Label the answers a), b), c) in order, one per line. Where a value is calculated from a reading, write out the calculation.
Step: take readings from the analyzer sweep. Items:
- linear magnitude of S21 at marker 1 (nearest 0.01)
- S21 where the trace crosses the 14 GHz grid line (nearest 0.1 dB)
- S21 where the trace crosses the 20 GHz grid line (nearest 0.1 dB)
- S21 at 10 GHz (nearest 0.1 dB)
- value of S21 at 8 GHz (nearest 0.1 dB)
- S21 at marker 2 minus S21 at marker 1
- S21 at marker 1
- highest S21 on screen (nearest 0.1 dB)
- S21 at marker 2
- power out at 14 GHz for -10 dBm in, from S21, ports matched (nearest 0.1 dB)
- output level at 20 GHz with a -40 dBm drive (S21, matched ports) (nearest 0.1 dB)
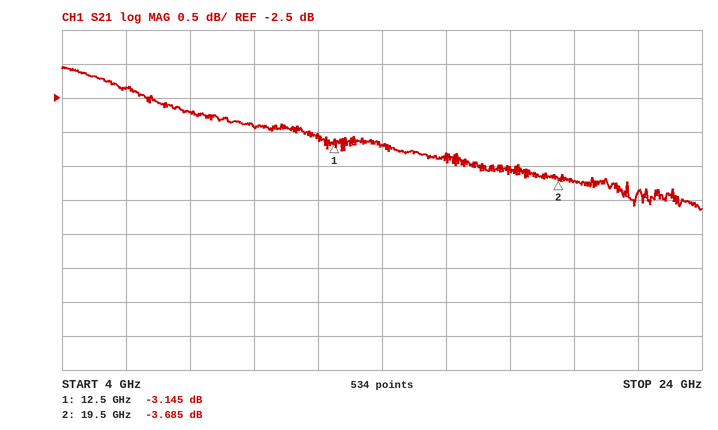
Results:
a) 10^(-3.145/20) ≈ 0.70
b) -3.2 dB
c) -3.7 dB
d) -2.9 dB
e) -2.7 dB
f) -3.685 − (-3.145) = -0.540 dB
g) -3.145 dB
h) -2.0 dB
i) -3.685 dB
j) -10 dBm + (-3.2 dB) = -13.2 dBm
k) -40 dBm + (-3.7 dB) = -43.7 dBm
